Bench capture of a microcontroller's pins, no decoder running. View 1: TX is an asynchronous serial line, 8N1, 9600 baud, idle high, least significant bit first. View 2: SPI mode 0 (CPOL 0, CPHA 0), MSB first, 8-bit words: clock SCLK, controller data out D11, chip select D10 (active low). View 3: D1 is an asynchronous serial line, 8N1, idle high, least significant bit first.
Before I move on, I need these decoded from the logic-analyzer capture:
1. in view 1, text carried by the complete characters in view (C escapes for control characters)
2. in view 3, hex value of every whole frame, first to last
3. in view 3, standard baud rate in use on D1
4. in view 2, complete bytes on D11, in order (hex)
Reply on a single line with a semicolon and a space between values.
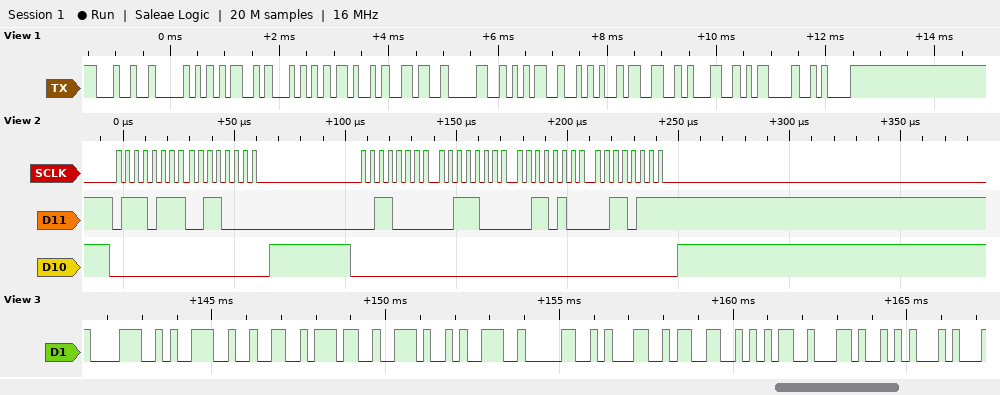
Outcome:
"$PMTK605*31\r\n"; 38 39 32 37 2E 39 30 31 33 35 2C 45; 4800 baud; 77 30 30 38 34 37
